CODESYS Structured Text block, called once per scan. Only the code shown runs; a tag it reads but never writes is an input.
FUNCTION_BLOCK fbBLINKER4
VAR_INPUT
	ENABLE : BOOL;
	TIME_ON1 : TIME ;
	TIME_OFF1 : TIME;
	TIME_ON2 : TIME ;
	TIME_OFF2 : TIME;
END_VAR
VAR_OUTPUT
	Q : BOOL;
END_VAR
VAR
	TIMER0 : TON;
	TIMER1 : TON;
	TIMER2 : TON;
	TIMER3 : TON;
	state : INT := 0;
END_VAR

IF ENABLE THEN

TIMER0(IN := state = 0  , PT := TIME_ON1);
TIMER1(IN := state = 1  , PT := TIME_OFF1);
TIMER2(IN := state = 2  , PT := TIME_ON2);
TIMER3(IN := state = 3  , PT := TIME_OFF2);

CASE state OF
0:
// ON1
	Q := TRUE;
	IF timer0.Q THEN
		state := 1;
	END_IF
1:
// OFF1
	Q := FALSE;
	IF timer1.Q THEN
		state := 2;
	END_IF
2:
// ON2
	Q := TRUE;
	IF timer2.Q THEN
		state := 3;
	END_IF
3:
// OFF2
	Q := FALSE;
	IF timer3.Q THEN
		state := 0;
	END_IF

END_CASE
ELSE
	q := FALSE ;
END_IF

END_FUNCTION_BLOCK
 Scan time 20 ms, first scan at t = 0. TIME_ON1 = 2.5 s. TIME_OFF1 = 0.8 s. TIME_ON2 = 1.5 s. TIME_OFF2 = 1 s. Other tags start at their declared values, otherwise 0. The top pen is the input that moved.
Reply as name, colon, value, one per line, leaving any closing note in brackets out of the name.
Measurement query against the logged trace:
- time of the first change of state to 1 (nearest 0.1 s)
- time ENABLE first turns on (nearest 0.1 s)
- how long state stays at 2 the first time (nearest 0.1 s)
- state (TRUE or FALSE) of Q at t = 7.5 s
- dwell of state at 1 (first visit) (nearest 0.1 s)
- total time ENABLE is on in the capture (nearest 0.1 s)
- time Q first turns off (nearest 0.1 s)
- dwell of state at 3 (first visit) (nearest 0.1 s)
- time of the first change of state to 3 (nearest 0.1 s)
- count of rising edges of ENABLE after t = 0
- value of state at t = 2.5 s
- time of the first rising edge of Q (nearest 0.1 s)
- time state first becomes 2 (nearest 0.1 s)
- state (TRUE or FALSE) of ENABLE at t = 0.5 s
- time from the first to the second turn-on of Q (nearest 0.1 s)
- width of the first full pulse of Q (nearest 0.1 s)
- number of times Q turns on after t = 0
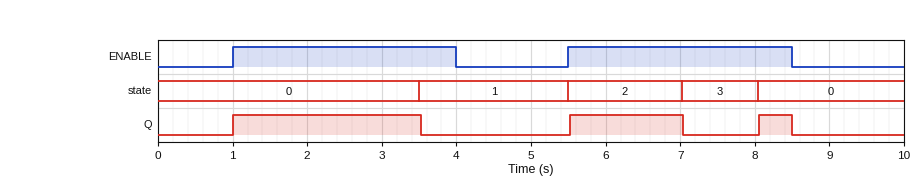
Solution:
time of the first change of state to 1: 3.5 s
time ENABLE first turns on: 1.0 s
how long state stays at 2 the first time: 1.5 s
state (TRUE or FALSE) of Q at t = 7.5 s: FALSE
dwell of state at 1 (first visit): 2.0 s
total time ENABLE is on in the capture: 6.0 s
time Q first turns off: 3.5 s
dwell of state at 3 (first visit): 1.0 s
time of the first change of state to 3: 7.0 s
count of rising edges of ENABLE after t = 0: 2
value of state at t = 2.5 s: 0
time of the first rising edge of Q: 1.0 s
time state first becomes 2: 5.5 s
state (TRUE or FALSE) of ENABLE at t = 0.5 s: FALSE
time from the first to the second turn-on of Q: 4.5 s
width of the first full pulse of Q: 2.5 s
number of times Q turns on after t = 0: 3
